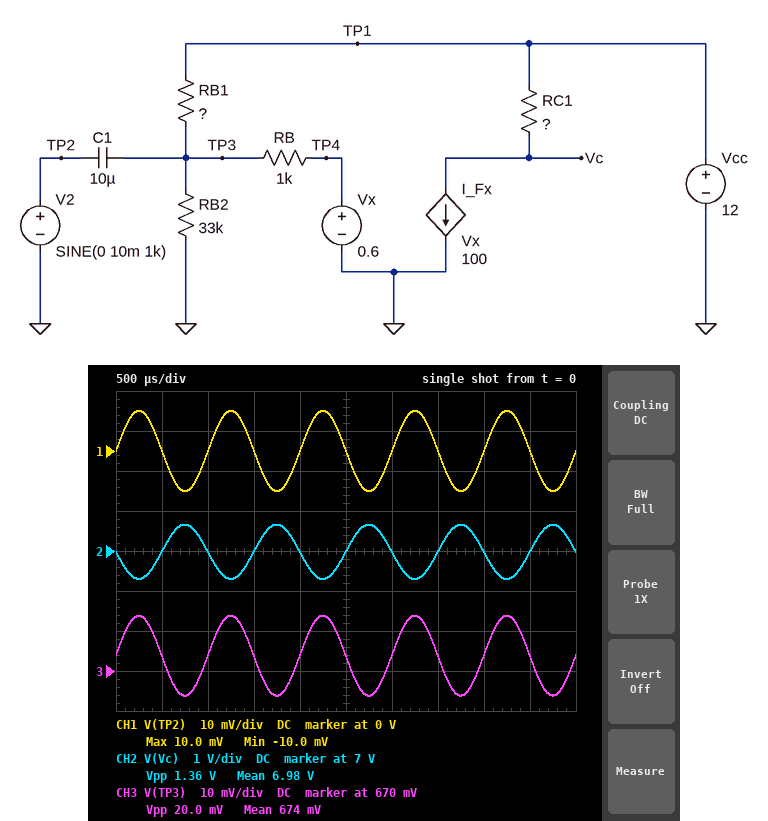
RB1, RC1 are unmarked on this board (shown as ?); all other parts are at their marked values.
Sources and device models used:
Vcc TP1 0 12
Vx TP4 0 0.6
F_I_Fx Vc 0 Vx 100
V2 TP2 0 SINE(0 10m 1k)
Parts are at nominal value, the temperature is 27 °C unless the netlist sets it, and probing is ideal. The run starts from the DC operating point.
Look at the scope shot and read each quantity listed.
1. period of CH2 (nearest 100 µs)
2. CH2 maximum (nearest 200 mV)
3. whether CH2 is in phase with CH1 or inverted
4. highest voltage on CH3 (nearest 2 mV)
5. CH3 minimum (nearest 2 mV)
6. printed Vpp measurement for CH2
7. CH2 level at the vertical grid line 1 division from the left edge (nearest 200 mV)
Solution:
1.0 ms
7.6 V
inverted
684 mV
664 mV
1.36 V
7.0 V
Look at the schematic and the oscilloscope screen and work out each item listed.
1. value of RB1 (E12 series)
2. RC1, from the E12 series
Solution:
120 kΩ
680 Ω
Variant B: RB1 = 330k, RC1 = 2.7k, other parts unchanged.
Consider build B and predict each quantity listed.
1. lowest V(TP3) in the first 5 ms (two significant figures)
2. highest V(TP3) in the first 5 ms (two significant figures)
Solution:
610 mV
630 mV
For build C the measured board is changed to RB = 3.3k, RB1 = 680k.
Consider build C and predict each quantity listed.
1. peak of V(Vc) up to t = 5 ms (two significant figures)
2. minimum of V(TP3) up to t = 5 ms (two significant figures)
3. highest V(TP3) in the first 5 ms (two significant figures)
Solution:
12 V
590 mV
610 mV
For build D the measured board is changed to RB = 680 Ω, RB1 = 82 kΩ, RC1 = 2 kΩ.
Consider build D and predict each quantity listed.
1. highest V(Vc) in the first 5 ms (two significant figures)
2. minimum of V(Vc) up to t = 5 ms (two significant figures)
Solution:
-8.5 V
-14 V
